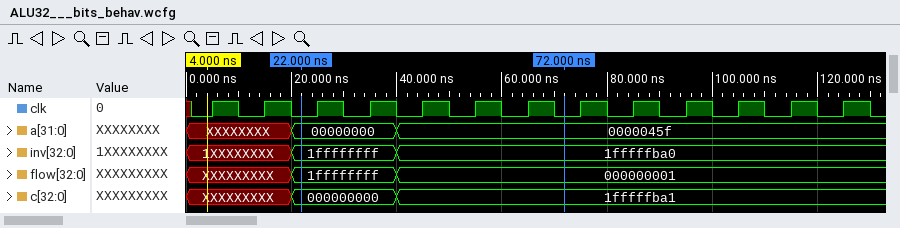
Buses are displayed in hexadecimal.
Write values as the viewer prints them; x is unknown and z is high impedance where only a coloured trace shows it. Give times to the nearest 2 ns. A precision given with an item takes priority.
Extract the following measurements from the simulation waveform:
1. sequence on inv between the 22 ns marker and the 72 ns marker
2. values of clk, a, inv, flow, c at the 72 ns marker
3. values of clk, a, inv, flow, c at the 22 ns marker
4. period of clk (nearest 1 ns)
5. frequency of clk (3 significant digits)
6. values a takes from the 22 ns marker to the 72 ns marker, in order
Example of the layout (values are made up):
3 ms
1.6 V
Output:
1ffffffff, 1fffffba0
clk=0, a=0000045f, inv=1fffffba0, flow=000000001, c=1fffffba1
clk=0, a=00000000, inv=1ffffffff, flow=1ffffffff, c=000000000
10 ns
100 MHz
00000000, 0000045f
